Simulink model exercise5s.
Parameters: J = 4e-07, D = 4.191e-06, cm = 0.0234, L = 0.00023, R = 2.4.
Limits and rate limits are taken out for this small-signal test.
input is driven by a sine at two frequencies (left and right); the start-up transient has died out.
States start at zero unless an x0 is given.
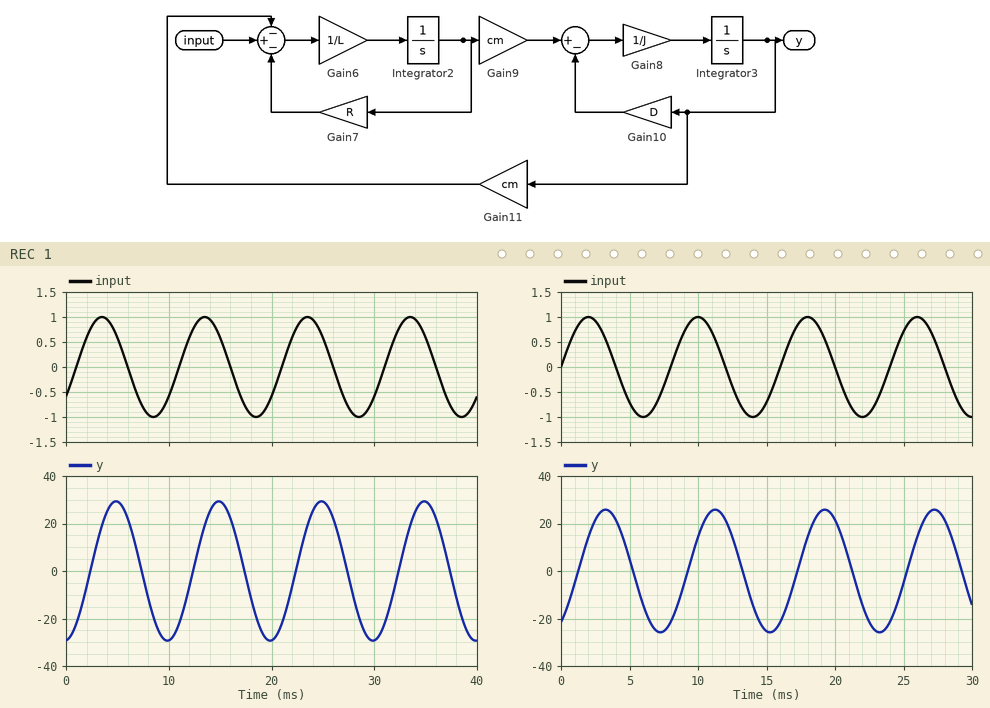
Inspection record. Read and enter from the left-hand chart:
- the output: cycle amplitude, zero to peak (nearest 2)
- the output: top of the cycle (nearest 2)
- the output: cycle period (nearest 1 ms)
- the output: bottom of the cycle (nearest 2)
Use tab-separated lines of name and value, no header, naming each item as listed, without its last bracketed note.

the output: cycle amplitude, zero to peak	30
the output: top of the cycle	30
the output: cycle period	10 ms
the output: bottom of the cycle	-30
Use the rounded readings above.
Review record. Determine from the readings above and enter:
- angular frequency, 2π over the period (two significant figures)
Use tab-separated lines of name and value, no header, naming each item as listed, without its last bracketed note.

angular frequency, 2π over the period	0.63 rad/ms
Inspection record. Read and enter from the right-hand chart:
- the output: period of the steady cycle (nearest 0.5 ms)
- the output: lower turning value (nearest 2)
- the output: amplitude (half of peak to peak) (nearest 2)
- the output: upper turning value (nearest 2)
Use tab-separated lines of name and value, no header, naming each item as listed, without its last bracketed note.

the output: period of the steady cycle	8.0 ms
the output: lower turning value	-26
the output: amplitude (half of peak to peak)	26
the output: upper turning value	26
